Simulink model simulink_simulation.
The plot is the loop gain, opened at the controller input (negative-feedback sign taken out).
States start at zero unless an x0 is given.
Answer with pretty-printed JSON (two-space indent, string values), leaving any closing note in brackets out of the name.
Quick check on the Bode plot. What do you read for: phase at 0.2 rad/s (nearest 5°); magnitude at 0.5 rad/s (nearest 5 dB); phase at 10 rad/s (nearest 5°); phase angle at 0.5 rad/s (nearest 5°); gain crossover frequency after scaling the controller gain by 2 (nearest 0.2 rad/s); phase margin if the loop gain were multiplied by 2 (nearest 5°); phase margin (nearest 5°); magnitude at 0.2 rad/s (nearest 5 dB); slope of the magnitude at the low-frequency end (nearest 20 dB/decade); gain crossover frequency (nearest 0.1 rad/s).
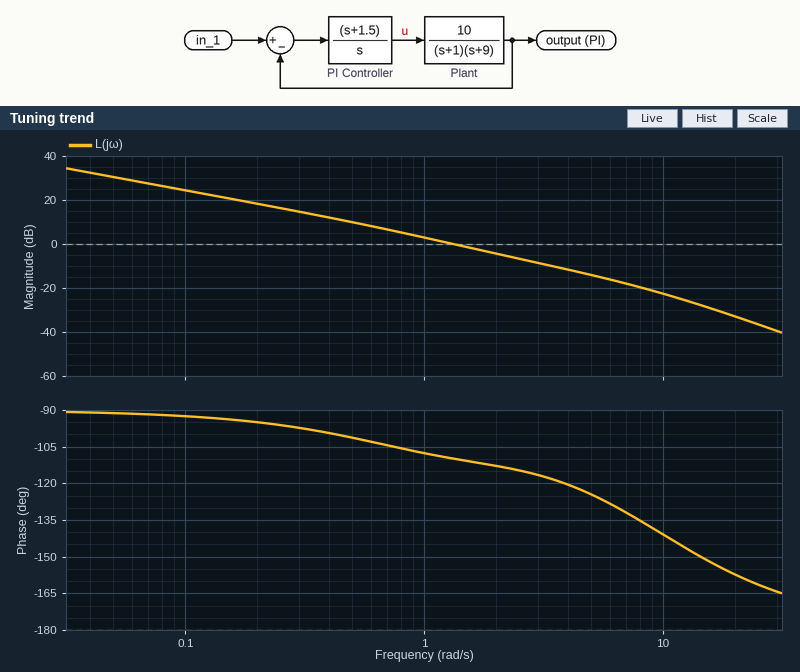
{
  "phase at 0.2 rad/s": "-95°",
  "magnitude at 0.5 rad/s": "10 dB",
  "phase at 10 rad/s": "-140°",
  "phase angle at 0.5 rad/s": "-100°",
  "gain crossover frequency after scaling the controller gain by 2": "2.4 rad/s",
  "phase margin if the loop gain were multiplied by 2": "65°",
  "phase margin": "70°",
  "magnitude at 0.2 rad/s": "20 dB",
  "slope of the magnitude at the low-frequency end": "-20 dB/decade",
  "gain crossover frequency": "1.3 rad/s"
}
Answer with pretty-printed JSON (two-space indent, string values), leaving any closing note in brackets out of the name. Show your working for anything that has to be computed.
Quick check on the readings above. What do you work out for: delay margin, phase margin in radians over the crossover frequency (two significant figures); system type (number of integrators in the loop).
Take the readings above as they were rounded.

{
  "delay margin, phase margin in radians over the crossover frequency": "70 × π / 180 / 1.3 = 0.94 s",
  "system type": "1"
}
